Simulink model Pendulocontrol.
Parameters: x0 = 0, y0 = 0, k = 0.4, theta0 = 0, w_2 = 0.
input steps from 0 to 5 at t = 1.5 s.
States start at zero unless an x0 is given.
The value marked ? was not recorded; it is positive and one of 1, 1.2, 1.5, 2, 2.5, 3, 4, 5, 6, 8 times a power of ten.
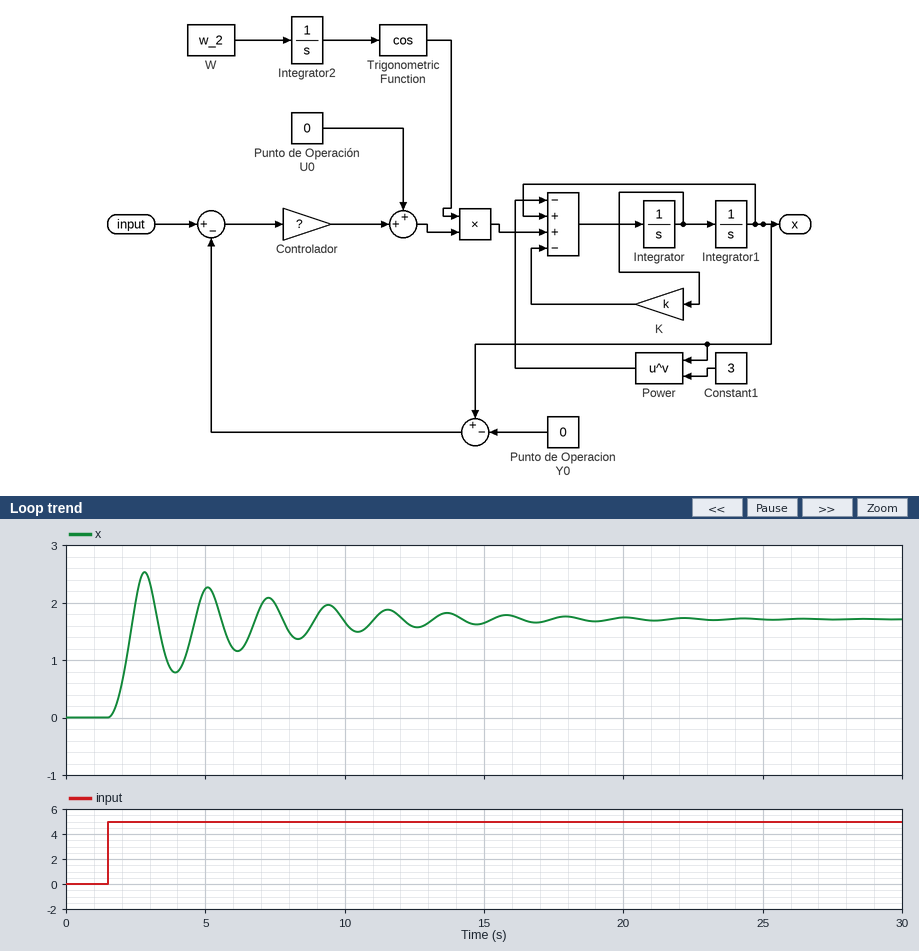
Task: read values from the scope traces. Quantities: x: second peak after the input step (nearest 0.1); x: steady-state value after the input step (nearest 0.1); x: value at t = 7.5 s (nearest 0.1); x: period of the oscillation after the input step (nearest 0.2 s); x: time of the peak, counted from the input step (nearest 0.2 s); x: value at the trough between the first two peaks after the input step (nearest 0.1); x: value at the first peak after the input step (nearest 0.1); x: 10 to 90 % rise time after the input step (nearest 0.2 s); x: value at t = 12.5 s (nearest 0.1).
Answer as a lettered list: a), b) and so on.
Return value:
a) 2.3
b) 1.7
c) 2.0
d) 2.2 s
e) 1.4 s
f) 0.8
g) 2.5
h) 0.6 s
i) 1.6
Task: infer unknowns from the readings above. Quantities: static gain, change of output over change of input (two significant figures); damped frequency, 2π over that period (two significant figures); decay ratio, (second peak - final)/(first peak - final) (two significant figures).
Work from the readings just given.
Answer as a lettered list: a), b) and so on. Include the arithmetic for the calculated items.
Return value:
a) (1.7 - 0) / (5 - 0) = 0.34
b) 2π / 2.2 = 2.9 rad/s
c) (2.3 - 1.7) / (2.5 - 1.7) = 0.75
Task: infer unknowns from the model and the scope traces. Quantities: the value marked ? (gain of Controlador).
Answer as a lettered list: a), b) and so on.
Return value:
a) 1
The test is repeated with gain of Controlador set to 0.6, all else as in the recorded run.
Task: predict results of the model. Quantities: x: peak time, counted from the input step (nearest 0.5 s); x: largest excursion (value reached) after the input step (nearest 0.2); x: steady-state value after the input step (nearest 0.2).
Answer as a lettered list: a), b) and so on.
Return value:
a) 1.5 s
b) 2.2
c) 1.6
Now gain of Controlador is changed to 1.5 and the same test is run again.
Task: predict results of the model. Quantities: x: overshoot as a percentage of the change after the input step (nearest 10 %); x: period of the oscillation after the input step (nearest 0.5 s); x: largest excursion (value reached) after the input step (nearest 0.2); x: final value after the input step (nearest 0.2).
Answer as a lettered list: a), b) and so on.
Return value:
a) 50 %
b) 2.0 s
c) 2.8
d) 1.8
